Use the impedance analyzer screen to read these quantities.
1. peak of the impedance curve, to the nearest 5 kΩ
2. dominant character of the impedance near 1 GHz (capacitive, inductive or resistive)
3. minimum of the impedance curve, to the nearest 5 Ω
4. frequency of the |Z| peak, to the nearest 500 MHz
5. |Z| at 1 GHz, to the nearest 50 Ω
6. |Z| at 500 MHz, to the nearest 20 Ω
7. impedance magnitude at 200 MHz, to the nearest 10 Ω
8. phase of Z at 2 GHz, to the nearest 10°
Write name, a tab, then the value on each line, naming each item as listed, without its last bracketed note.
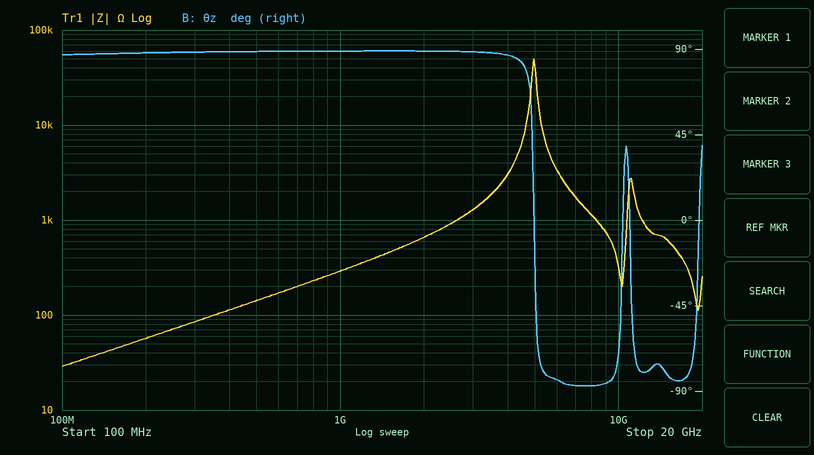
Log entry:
peak of the impedance curve, to the nearest 5 kΩ	50 kΩ
dominant character of the impedance near 1 GHz	inductive
minimum of the impedance curve, to the nearest 5 Ω	30 Ω
frequency of the |Z| peak, to the nearest 500 MHz	5.0 GHz
|Z| at 1 GHz, to the nearest 50 Ω	300 Ω
|Z| at 500 MHz, to the nearest 20 Ω	140 Ω
impedance magnitude at 200 MHz, to the nearest 10 Ω	60 Ω
phase of Z at 2 GHz, to the nearest 10°	90°
